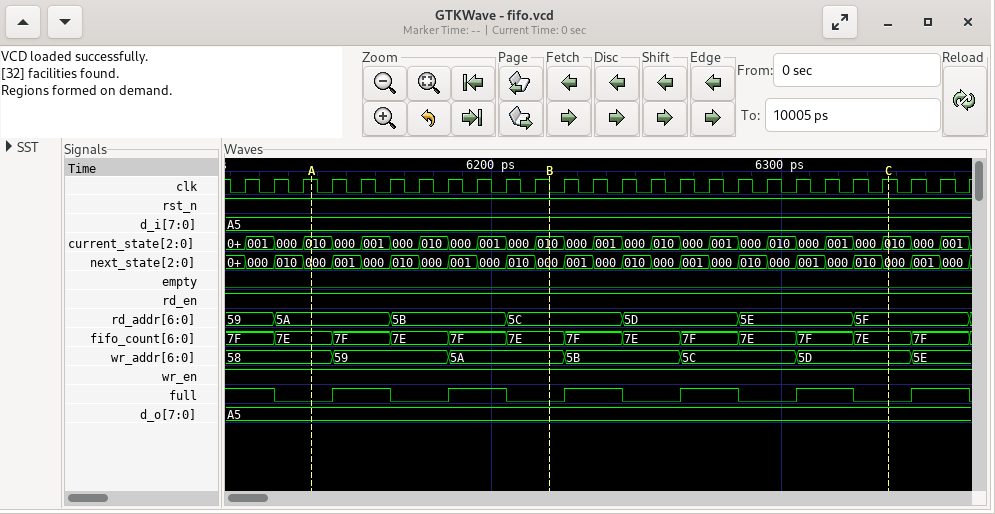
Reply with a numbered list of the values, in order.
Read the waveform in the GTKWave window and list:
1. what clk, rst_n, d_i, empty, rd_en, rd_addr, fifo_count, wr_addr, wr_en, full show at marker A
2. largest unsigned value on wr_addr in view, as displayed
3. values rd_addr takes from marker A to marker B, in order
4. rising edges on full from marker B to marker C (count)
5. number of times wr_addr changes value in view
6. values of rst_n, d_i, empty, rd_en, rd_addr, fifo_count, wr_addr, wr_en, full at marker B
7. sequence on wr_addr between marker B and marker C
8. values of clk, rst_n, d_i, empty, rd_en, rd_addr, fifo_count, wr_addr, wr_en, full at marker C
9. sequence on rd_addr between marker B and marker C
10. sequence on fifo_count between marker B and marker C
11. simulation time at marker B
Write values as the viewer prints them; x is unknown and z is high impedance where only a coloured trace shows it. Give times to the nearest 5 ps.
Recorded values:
1. clk=1, rst_n=1, d_i=A5, empty=0, rd_en=1, rd_addr=5A, fifo_count=7E, wr_addr=58, wr_en=1, full=0
2. 5E
3. 5A, 5B, 5C
4. 3
5. 6
6. rst_n=1, d_i=A5, empty=0, rd_en=1, rd_addr=5C, fifo_count=7E, wr_addr=5A, wr_en=1, full=0
7. 5A, 5B, 5C, 5D
8. clk=1, rst_n=1, d_i=A5, empty=0, rd_en=1, rd_addr=5F, fifo_count=7E, wr_addr=5D, wr_en=1, full=0
9. 5C, 5D, 5E, 5F
10. 7E, 7F, 7E, 7F, 7E, 7F, 7E
11. 6220 ps
